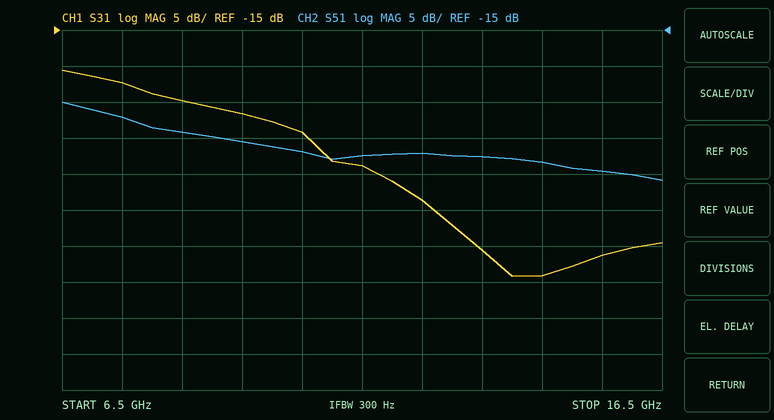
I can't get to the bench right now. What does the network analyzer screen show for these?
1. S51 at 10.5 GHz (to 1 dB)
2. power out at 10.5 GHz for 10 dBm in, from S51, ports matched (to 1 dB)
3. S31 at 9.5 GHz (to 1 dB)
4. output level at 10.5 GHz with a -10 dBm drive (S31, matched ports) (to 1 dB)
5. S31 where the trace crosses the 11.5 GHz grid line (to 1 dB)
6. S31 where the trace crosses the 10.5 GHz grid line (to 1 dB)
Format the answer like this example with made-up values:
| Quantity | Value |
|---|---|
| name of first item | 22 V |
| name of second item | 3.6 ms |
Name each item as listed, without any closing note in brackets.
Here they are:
| Quantity | Value |
|---|---|
| S51 at 10.5 GHz | -32 dB |
| power out at 10.5 GHz for 10 dBm in, from S51, ports matched | -22 dBm |
| S31 at 9.5 GHz | -27 dB |
| output level at 10.5 GHz with a -10 dBm drive (S31, matched ports) | -39 dBm |
| S31 where the trace crosses the 11.5 GHz grid line | -34 dB |
| S31 where the trace crosses the 10.5 GHz grid line | -29 dB |
